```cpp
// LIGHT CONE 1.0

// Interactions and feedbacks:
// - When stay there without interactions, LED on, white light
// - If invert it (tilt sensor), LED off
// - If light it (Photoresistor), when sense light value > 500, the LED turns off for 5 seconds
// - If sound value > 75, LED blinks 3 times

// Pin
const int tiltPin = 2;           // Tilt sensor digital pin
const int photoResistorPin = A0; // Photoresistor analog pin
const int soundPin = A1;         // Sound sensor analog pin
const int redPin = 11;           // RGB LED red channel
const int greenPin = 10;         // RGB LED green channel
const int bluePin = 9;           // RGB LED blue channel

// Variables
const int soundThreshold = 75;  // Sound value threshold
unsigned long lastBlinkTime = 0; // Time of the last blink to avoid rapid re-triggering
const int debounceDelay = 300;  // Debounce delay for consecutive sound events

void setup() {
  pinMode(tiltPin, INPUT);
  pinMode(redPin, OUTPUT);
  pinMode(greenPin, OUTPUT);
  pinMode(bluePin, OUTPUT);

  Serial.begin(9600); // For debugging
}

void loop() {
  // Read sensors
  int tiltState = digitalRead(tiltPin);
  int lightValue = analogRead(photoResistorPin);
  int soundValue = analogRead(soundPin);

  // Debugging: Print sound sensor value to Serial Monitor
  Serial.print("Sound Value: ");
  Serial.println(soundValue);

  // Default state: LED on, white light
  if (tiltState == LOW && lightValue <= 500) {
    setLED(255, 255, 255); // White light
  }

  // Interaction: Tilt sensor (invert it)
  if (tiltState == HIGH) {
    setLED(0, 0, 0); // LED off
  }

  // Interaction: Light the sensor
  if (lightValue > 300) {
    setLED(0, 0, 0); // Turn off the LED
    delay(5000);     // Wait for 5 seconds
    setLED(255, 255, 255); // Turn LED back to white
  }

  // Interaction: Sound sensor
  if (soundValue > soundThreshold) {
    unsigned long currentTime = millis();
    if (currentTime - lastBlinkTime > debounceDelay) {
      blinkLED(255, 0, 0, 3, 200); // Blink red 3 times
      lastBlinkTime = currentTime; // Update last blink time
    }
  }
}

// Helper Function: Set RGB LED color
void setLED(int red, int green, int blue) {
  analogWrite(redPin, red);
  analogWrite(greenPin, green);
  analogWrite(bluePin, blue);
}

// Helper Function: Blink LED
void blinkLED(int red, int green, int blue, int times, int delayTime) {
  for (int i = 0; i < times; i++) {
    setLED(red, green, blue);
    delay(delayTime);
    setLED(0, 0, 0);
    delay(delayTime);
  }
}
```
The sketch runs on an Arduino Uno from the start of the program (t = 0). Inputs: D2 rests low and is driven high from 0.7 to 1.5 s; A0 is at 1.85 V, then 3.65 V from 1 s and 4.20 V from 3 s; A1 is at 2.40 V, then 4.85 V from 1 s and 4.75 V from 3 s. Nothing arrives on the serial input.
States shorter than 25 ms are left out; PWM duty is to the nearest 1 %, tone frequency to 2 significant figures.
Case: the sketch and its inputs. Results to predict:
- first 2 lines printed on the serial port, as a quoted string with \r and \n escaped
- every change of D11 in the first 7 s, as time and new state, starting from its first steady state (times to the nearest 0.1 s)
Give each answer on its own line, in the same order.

"Sound Value: 491\r\nSound Value: 972\r\n"
0 s low; 5 s high; 5.2 s low; 5.4 s high; 5.6 s low; 5.8 s high; 6 s low
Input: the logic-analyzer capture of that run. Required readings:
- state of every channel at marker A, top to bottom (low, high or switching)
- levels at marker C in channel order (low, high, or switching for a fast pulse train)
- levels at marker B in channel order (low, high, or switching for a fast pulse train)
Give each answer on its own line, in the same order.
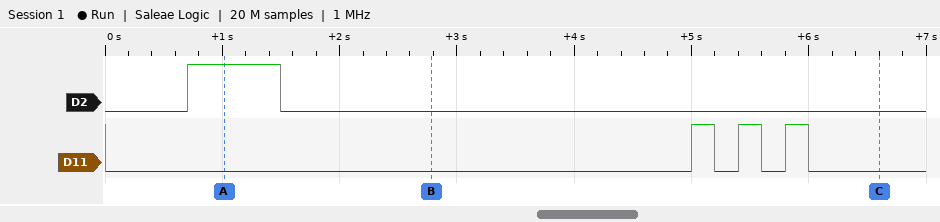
D2 high, D11 low
D2 low, D11 low
D2 low, D11 low
